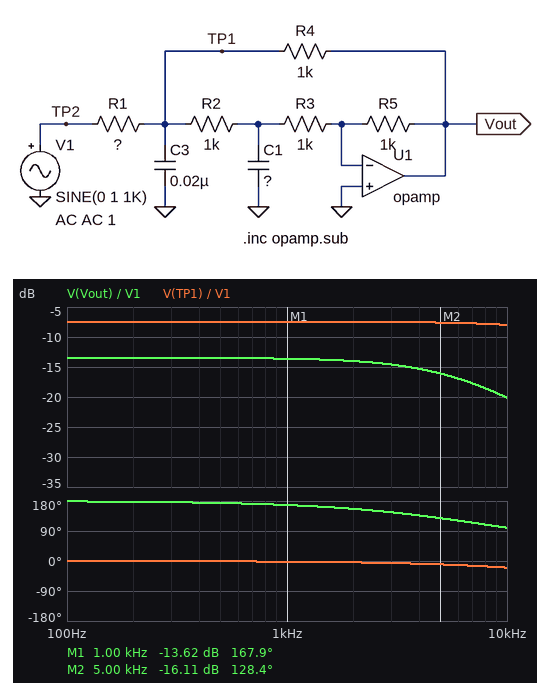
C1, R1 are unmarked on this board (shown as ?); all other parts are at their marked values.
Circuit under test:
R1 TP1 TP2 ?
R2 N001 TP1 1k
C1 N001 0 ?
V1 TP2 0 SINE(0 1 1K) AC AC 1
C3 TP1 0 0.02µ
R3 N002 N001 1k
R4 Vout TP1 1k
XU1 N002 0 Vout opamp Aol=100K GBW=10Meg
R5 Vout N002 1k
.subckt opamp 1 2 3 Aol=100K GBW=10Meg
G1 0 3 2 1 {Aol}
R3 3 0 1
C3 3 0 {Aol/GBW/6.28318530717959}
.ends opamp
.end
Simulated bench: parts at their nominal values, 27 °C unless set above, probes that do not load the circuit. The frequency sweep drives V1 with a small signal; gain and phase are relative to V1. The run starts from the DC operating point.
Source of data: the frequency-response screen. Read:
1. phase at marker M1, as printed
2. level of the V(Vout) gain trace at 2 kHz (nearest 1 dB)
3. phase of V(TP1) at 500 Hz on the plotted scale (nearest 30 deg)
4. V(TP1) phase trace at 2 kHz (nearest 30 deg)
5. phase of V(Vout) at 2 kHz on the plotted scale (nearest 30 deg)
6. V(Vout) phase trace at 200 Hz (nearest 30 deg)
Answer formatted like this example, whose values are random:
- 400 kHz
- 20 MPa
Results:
- 167.9 deg
- -14 dB
- 0 deg
- 0 deg
- 150 deg
- 180 deg
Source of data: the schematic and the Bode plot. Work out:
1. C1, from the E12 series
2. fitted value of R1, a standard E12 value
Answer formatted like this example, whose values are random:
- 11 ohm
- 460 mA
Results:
- 56 nF
- 680 Ω
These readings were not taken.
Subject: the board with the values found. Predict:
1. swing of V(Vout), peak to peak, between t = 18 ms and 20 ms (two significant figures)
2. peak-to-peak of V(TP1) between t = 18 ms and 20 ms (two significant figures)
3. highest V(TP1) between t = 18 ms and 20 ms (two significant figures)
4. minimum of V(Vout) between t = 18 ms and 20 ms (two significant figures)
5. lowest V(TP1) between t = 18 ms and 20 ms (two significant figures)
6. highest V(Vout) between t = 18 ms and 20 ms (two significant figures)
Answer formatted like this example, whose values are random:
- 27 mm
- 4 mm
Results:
- 420 mV
- 850 mV
- 420 mV
- -210 mV
- -420 mV
- 210 mV
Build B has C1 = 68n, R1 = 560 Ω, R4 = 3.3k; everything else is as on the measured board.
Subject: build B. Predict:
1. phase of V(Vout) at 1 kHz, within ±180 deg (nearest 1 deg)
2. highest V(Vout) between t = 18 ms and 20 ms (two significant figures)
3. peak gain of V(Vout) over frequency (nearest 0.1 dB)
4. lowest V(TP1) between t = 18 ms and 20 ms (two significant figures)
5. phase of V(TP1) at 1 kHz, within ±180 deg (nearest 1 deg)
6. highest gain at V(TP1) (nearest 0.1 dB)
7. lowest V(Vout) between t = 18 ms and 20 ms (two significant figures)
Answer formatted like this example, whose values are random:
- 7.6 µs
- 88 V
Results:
- 164 deg
- 320 mV
- -9.7 dB
- -650 mV
- -4 deg
- -3.7 dB
- -320 mV
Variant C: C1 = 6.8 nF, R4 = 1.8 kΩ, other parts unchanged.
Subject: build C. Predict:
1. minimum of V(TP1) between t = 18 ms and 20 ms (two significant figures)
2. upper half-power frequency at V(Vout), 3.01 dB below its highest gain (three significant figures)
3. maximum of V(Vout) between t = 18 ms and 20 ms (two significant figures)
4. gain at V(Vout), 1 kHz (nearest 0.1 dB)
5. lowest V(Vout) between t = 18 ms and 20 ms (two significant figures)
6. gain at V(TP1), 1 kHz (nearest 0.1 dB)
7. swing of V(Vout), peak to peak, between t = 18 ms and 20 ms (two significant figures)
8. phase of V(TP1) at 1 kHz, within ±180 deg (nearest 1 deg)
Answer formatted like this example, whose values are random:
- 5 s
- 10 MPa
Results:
- -520 mV
- 18.3 kHz
- 260 mV
- -11.6 dB
- -260 mV
- -5.6 dB
- 520 mV
- -3 deg
